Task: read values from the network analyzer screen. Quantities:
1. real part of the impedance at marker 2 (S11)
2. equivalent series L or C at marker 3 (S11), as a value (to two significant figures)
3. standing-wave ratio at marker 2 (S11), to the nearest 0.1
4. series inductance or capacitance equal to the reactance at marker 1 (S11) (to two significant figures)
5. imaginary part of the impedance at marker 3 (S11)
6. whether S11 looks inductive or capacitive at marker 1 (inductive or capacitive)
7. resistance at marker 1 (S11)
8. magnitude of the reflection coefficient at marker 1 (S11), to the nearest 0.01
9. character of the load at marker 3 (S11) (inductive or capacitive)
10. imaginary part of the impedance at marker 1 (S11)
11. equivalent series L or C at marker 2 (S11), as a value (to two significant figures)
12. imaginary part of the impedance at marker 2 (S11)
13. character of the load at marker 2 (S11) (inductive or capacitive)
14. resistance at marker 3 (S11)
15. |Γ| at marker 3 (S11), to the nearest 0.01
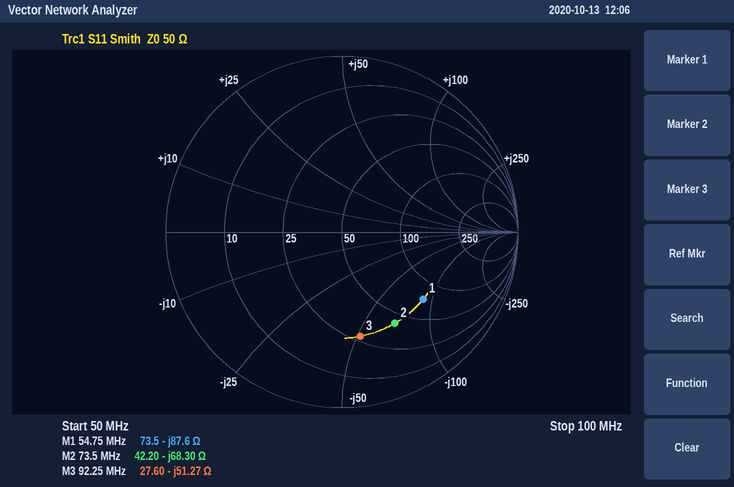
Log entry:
42.20 Ω
34 pF
4.0
33 pF
-51.27 Ω
capacitive
73.5 Ω
0.60
capacitive
-87.6 Ω
32 pF
-68.30 Ω
capacitive
27.60 Ω
0.60
